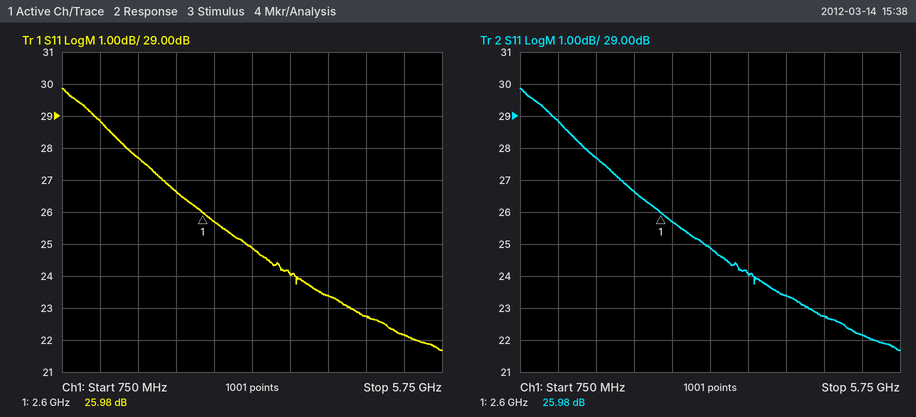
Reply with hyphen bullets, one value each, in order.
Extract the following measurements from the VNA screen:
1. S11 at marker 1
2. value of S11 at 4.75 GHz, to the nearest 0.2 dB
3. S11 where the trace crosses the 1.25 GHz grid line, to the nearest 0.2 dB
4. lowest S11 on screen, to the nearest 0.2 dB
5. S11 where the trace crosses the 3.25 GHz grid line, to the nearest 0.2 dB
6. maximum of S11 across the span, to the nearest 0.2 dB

- 25.98 dB
- 22.8 dB
- 28.8 dB
- 21.6 dB
- 24.8 dB
- 29.8 dB
